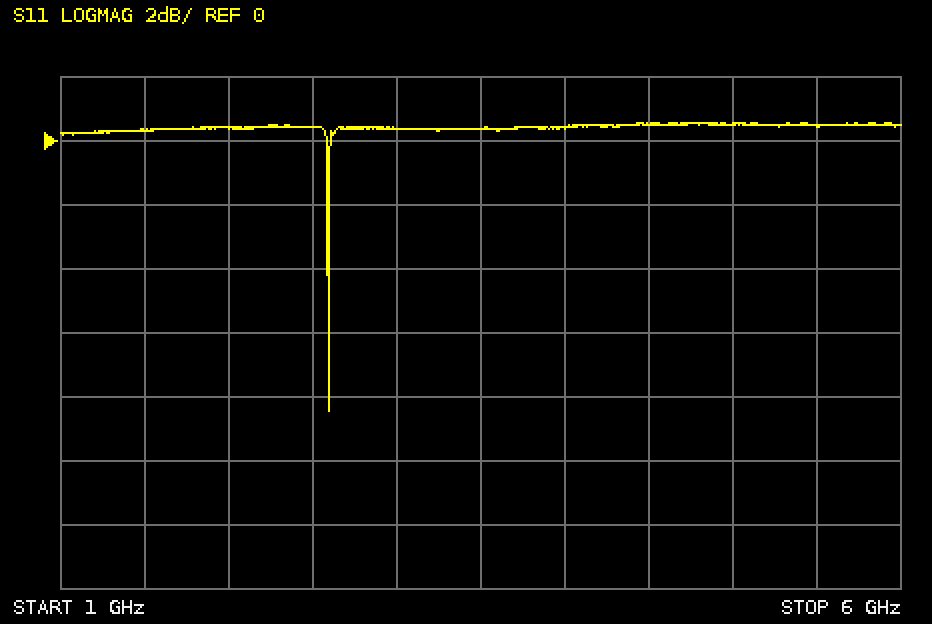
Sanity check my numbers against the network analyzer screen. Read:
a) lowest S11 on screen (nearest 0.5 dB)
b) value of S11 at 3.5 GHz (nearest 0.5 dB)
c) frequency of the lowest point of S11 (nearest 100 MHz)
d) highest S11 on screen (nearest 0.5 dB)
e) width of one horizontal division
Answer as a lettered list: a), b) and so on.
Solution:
a) -8.5 dB
b) 0.5 dB
c) 2.6 GHz
d) 0.5 dB
e) 500 MHz
